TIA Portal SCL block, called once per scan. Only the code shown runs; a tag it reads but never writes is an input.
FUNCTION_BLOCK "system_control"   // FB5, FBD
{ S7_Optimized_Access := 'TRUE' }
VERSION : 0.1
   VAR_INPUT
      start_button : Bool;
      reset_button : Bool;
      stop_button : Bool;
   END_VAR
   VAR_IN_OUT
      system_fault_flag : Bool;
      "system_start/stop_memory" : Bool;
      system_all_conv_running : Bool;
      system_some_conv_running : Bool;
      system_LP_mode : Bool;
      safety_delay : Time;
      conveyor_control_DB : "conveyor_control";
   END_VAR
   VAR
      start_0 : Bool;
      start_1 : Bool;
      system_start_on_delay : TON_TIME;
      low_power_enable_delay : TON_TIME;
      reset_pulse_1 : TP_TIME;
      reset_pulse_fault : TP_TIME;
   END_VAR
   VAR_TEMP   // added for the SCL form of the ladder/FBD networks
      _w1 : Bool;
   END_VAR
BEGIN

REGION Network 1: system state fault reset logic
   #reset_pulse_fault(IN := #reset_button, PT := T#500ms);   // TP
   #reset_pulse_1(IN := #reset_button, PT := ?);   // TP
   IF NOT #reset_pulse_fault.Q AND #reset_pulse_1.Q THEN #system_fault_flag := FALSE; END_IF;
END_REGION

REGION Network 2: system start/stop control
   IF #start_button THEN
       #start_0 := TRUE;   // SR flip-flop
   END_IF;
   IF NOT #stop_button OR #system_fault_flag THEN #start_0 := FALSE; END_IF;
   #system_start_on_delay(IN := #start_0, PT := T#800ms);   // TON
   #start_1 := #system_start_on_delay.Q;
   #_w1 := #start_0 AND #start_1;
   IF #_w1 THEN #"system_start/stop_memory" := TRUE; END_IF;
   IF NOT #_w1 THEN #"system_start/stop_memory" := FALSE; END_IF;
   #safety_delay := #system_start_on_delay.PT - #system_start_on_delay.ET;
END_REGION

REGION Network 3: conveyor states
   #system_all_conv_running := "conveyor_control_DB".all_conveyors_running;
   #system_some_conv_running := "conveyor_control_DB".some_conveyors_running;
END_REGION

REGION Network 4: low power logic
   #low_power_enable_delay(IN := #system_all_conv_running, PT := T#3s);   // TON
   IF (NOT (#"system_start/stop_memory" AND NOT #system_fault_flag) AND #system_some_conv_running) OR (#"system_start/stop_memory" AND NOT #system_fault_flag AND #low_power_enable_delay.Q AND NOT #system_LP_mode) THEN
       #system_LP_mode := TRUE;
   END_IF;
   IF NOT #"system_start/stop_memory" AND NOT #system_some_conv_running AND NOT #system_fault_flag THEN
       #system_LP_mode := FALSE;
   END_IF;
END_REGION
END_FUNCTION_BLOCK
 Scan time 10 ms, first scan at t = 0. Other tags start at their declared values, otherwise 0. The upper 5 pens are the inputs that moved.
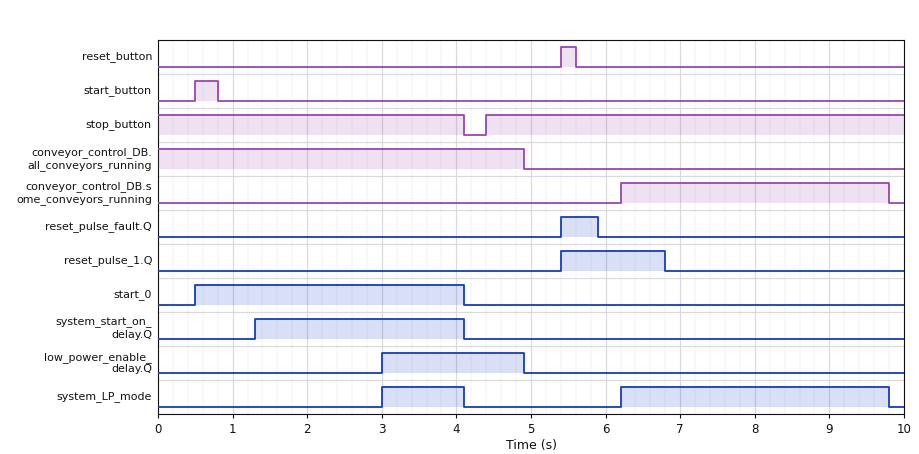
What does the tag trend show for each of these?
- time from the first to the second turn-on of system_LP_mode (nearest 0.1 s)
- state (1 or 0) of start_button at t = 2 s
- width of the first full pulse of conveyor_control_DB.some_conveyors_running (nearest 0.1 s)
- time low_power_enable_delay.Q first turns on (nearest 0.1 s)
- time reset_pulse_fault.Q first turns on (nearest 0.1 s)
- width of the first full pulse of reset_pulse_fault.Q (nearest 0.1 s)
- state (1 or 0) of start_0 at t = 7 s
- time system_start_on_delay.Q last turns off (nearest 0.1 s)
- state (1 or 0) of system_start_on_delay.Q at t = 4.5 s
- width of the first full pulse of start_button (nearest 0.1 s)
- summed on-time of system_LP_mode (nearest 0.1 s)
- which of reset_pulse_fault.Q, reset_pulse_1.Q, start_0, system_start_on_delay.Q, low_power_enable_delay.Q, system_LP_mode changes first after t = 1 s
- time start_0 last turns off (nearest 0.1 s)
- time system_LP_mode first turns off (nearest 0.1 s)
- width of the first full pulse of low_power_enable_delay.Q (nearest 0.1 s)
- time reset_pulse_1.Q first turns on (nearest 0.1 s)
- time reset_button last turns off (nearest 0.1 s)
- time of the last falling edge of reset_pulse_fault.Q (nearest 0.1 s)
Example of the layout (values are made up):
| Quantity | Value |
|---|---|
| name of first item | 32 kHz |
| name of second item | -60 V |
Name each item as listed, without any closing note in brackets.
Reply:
| Quantity | Value |
|---|---|
| time from the first to the second turn-on of system_LP_mode | 3.2 s |
| state (1 or 0) of start_button at t = 2 s | 0 |
| width of the first full pulse of conveyor_control_DB.some_conveyors_running | 3.6 s |
| time low_power_enable_delay.Q first turns on | 3.0 s |
| time reset_pulse_fault.Q first turns on | 5.4 s |
| width of the first full pulse of reset_pulse_fault.Q | 0.5 s |
| state (1 or 0) of start_0 at t = 7 s | 0 |
| time system_start_on_delay.Q last turns off | 4.1 s |
| state (1 or 0) of system_start_on_delay.Q at t = 4.5 s | 0 |
| width of the first full pulse of start_button | 0.3 s |
| summed on-time of system_LP_mode | 4.7 s |
| which of reset_pulse_fault.Q, reset_pulse_1.Q, start_0, system_start_on_delay.Q, low_power_enable_delay.Q, system_LP_mode changes first after t = 1 s | system_start_on_delay.Q |
| time start_0 last turns off | 4.1 s |
| time system_LP_mode first turns off | 4.1 s |
| width of the first full pulse of low_power_enable_delay.Q | 1.9 s |
| time reset_pulse_1.Q first turns on | 5.4 s |
| time reset_button last turns off | 5.6 s |
| time of the last falling edge of reset_pulse_fault.Q | 5.9 s |
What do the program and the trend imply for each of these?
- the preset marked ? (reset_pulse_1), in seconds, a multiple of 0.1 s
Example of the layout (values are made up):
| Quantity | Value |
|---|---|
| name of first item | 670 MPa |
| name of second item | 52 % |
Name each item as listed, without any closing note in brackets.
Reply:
| Quantity | Value |
|---|---|
| the preset marked ? (reset_pulse_1), in seconds, a multiple of 0.1 s | 1.4 s |
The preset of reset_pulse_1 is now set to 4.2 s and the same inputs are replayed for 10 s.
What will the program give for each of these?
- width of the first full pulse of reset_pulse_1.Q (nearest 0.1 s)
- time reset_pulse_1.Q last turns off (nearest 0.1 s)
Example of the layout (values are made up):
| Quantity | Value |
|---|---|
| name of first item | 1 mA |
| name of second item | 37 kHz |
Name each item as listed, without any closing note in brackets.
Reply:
| Quantity | Value |
|---|---|
| width of the first full pulse of reset_pulse_1.Q | 4.2 s |
| time reset_pulse_1.Q last turns off | 9.6 s |
